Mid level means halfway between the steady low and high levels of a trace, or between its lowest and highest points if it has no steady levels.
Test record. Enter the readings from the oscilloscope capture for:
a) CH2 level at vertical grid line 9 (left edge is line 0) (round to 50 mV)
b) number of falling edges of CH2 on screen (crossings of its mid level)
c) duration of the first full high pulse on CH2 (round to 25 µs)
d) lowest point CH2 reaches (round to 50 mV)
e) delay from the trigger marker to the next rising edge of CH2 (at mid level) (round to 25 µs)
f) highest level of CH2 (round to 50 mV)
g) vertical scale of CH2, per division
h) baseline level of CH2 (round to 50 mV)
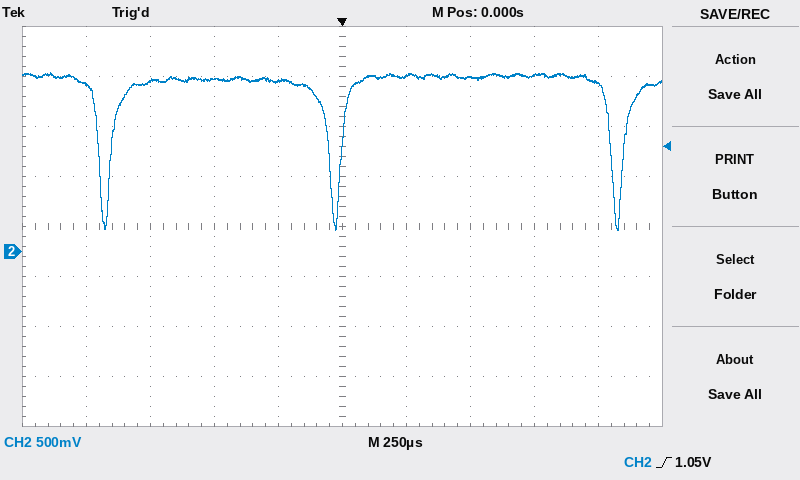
1.70 V
3
850 µs
200 mV
1.100 ms
1.80 V
500 mV
1.75 V
